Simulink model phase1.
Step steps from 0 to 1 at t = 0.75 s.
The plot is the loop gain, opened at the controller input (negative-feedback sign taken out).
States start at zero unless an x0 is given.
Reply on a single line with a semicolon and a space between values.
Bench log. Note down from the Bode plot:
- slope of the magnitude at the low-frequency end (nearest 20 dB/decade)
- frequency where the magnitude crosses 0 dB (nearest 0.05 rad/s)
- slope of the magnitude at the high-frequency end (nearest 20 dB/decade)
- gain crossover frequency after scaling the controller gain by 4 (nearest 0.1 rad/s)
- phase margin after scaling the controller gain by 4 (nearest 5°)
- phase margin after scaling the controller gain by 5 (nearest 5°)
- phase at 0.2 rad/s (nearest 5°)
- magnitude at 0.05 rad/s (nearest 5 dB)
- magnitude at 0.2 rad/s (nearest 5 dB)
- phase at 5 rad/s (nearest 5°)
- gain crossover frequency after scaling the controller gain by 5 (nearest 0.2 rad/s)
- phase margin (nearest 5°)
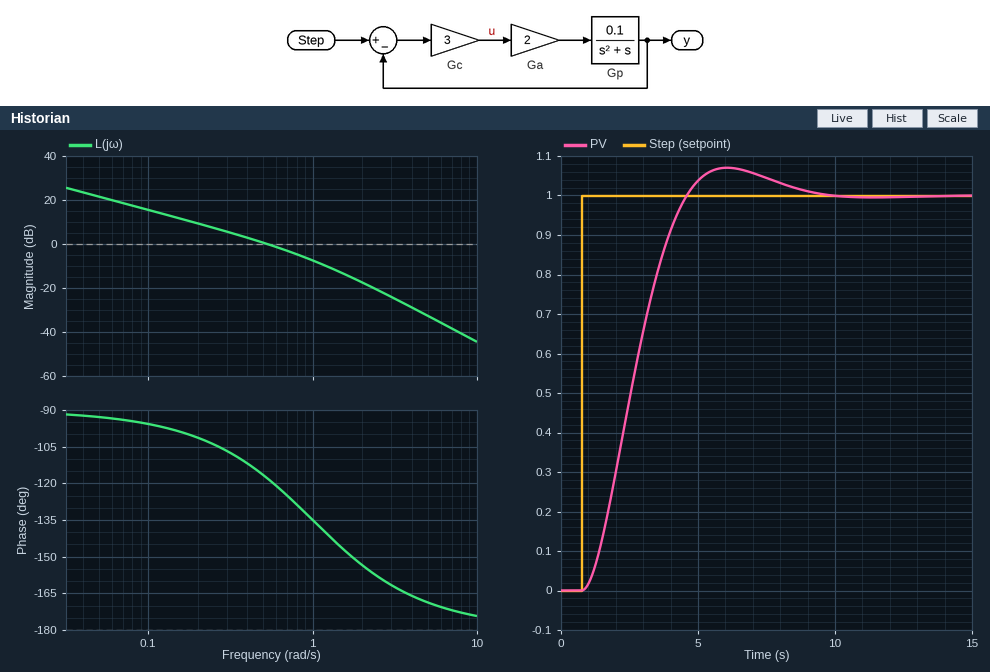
-20 dB/decade; 0.55 rad/s; -40 dB/decade; 1.4 rad/s; 35°; 30°; -100°; 20 dB; 10 dB; -170°; 1.6 rad/s; 60°
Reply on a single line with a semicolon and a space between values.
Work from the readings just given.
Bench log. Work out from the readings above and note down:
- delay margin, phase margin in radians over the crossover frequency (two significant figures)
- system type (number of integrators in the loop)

1.9 s; 1
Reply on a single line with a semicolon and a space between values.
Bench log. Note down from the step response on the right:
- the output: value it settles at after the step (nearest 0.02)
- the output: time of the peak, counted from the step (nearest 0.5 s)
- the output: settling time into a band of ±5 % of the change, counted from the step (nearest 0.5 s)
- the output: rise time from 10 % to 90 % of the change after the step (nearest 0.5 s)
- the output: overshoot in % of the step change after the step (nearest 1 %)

1.00; 5.5 s; 6.5 s; 2.5 s; 7 %
